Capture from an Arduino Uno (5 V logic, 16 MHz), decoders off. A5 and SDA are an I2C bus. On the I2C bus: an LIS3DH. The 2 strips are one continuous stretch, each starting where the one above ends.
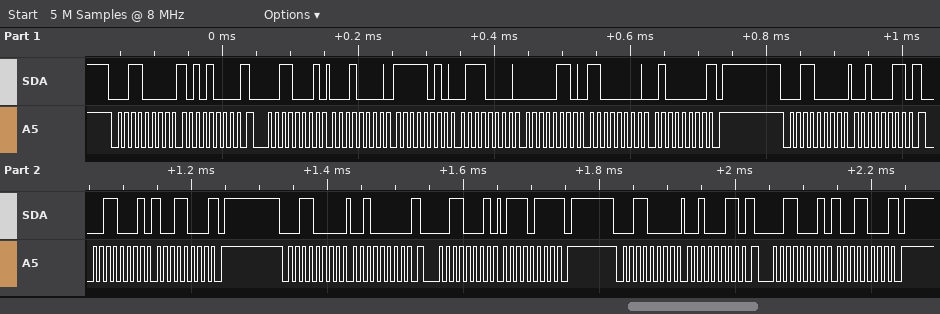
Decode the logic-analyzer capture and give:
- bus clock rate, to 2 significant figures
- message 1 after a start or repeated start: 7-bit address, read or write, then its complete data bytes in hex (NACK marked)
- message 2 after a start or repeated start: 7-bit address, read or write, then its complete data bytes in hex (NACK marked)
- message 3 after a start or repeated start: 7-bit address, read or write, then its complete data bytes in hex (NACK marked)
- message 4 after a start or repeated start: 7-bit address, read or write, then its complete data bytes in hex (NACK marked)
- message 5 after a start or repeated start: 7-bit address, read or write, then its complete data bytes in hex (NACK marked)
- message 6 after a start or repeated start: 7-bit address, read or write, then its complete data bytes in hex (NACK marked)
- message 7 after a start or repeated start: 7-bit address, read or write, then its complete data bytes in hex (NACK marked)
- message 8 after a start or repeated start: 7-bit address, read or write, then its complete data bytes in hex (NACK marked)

100 kHz
0x18 write: A8
0x18 read: 10 FA 70 06 C0 40 NACK
0x18 write: 23
0x18 read: 98 NACK
0x18 write: 20
0x18 read: 77 NACK
0x18 write: 23
0x18 read: 98 NACK
